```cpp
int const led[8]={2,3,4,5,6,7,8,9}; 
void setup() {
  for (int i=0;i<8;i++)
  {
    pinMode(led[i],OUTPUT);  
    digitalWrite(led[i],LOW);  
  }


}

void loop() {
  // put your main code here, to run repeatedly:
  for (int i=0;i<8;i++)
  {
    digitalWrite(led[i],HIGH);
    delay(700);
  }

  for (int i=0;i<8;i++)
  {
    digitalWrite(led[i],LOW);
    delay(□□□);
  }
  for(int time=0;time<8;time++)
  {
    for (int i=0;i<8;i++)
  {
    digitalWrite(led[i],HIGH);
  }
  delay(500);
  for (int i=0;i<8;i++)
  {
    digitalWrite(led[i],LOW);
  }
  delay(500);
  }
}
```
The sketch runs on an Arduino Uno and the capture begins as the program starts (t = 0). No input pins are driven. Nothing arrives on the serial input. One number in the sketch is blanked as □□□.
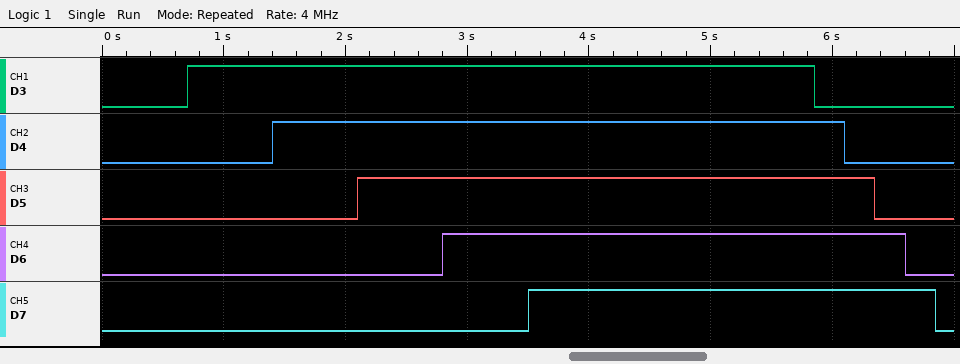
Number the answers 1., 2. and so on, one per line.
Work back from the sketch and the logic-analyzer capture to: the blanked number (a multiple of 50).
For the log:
1. 250
